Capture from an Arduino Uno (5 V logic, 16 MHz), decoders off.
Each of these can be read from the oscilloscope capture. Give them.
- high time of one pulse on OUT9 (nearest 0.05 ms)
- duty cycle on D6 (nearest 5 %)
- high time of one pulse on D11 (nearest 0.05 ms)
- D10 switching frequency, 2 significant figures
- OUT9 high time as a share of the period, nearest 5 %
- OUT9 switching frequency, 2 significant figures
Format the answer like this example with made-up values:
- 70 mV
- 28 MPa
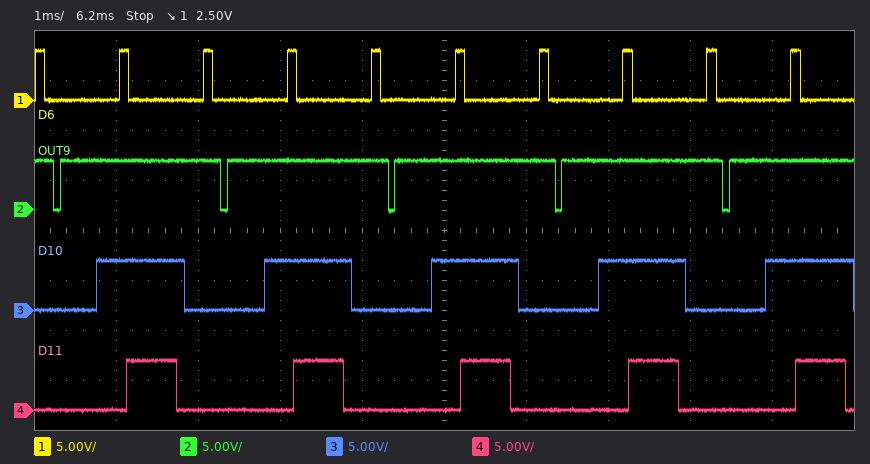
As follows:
- 1.95 ms
- 10 %
- 0.60 ms
- 490 Hz
- 95 %
- 490 Hz
